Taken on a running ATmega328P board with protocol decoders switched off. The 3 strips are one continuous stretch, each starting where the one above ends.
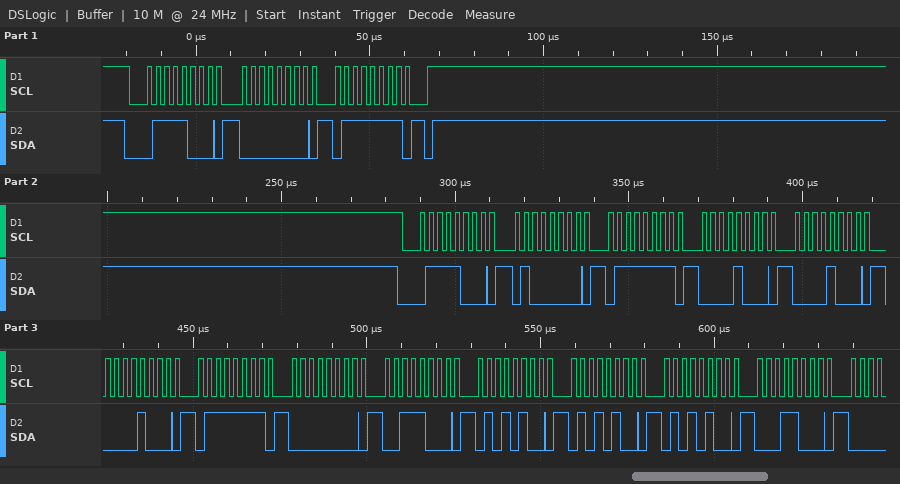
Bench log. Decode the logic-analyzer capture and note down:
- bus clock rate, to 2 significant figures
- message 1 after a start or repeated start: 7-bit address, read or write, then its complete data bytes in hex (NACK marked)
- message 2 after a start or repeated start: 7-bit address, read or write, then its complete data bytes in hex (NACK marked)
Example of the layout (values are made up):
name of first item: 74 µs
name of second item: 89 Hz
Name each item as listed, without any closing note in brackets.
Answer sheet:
bus clock rate, to 2 significant figures: 400 kHz
message 1 after a start or repeated start: 7-bit address, read or write, then its complete data bytes in hex: 0x3C write: 00 7F
message 2 after a start or repeated start: 7-bit address, read or write, then its complete data bytes in hex: 0x3C write: 40 7F 08 08 08 7F 00 38 54 54 54 18
